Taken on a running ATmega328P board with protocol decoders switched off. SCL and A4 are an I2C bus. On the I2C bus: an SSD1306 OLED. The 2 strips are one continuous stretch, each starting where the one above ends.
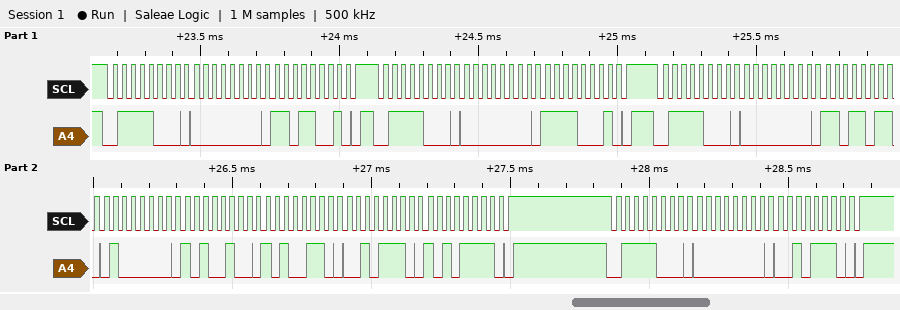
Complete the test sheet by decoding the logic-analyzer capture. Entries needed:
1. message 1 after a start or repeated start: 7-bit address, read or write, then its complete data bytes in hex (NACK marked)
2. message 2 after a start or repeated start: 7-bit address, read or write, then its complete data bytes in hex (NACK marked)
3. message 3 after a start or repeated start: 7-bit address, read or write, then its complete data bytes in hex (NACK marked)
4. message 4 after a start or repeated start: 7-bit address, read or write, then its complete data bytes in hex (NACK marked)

0x3C write: 00 D9
0x3C write: 00 F1
0x3C write: 00 DB 40 A4 A6 2E AF
0x3C write: 00 2E
